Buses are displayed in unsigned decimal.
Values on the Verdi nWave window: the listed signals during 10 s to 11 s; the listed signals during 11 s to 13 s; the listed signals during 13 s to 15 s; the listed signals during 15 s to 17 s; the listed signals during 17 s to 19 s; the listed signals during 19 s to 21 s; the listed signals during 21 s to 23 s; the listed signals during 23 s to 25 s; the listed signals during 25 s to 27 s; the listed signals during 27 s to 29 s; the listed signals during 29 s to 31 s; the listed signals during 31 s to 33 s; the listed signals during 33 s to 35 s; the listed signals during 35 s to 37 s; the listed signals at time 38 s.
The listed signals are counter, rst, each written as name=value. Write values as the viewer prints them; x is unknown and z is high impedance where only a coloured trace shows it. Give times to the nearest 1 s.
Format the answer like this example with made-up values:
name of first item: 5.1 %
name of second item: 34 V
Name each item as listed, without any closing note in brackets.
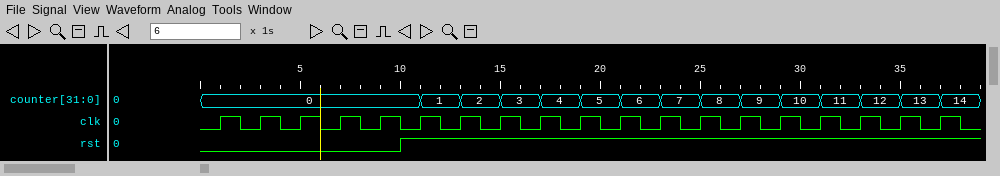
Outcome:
the listed signals during 10 s to 11 s: counter=0, rst=1
the listed signals during 11 s to 13 s: counter=1, rst=1
the listed signals during 13 s to 15 s: counter=2, rst=1
the listed signals during 15 s to 17 s: counter=3, rst=1
the listed signals during 17 s to 19 s: counter=4, rst=1
the listed signals during 19 s to 21 s: counter=5, rst=1
the listed signals during 21 s to 23 s: counter=6, rst=1
the listed signals during 23 s to 25 s: counter=7, rst=1
the listed signals during 25 s to 27 s: counter=8, rst=1
the listed signals during 27 s to 29 s: counter=9, rst=1
the listed signals during 29 s to 31 s: counter=10, rst=1
the listed signals during 31 s to 33 s: counter=11, rst=1
the listed signals during 33 s to 35 s: counter=12, rst=1
the listed signals during 35 s to 37 s: counter=13, rst=1
the listed signals at time 38 s: counter=14, rst=1
